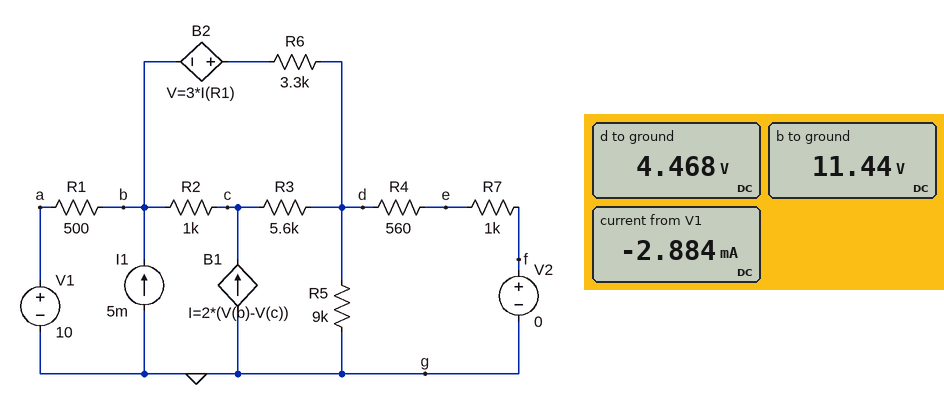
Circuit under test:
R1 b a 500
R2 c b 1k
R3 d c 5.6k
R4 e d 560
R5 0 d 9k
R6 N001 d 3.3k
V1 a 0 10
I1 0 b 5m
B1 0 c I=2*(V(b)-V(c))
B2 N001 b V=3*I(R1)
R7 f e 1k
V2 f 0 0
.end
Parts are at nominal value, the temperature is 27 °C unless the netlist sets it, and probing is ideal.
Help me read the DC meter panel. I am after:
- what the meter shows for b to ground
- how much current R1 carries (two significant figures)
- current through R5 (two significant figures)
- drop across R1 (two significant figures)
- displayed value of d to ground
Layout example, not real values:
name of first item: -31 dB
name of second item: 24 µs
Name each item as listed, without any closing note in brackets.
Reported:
what the meter shows for b to ground: 11.44 V
how much current R1 carries: 2.9 mA
current through R5: 500 µA
drop across R1: 1.4 V
displayed value of d to ground: 4.468 V
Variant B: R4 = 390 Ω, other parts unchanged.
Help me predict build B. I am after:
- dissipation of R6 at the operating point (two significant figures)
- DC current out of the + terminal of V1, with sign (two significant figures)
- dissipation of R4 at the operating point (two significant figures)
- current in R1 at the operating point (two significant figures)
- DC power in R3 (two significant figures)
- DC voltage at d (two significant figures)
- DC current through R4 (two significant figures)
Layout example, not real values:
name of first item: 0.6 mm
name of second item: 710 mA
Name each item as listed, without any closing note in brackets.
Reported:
dissipation of R6 at the operating point: 16 mW
DC current out of the + terminal of V1, with sign: -2.8 mA
dissipation of R4 at the operating point: 3.5 mW
current in R1 at the operating point: 2.8 mA
DC power in R3: 9.3 mW
DC voltage at d: 4.2 V
DC current through R4: 3.0 mA
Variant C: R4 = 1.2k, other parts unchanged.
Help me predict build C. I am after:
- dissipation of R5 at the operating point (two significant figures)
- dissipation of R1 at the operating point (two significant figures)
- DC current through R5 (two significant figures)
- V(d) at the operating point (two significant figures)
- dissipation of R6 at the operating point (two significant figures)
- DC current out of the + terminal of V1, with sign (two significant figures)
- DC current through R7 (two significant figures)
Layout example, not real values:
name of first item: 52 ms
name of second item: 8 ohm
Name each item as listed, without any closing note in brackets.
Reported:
dissipation of R5 at the operating point: 3.1 mW
dissipation of R1 at the operating point: 4.8 mW
DC current through R5: 590 µA
V(d) at the operating point: 5.3 V
dissipation of R6 at the operating point: 12 mW
DC current out of the + terminal of V1, with sign: -3.1 mA
DC current through R7: 2.4 mA
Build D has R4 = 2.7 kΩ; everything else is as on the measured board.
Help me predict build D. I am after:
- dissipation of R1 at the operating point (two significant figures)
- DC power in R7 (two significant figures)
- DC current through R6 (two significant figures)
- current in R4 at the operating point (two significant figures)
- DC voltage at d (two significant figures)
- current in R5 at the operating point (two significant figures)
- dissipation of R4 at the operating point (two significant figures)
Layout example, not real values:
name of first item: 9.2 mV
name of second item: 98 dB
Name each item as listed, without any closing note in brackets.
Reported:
dissipation of R1 at the operating point: 5.9 mW
DC power in R7: 3.1 mW
DC current through R6: 1.6 mA
current in R4 at the operating point: 1.8 mA
DC voltage at d: 6.5 V
current in R5 at the operating point: 730 µA
dissipation of R4 at the operating point: 8.4 mW
